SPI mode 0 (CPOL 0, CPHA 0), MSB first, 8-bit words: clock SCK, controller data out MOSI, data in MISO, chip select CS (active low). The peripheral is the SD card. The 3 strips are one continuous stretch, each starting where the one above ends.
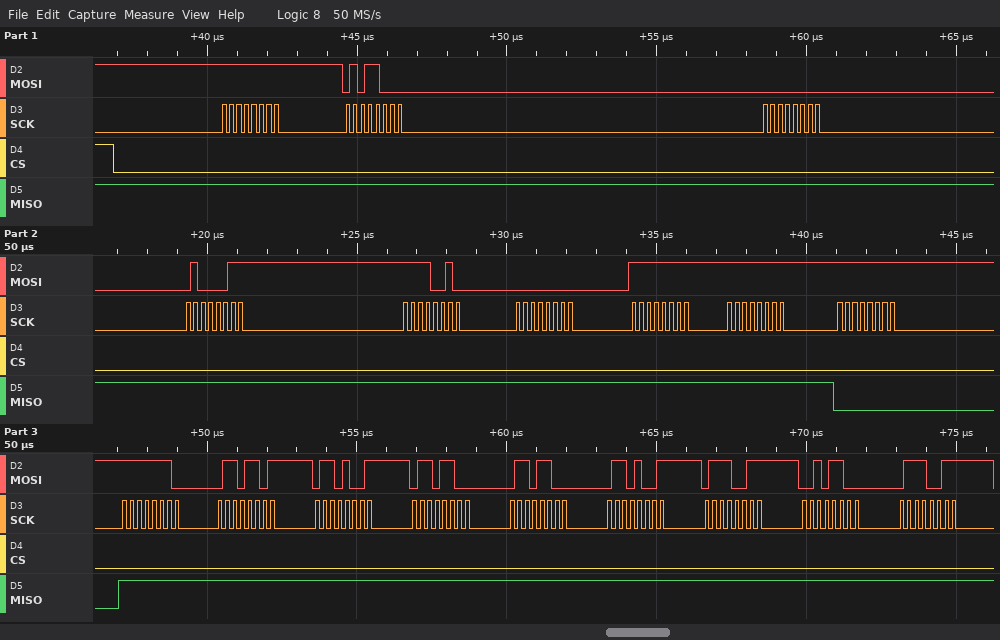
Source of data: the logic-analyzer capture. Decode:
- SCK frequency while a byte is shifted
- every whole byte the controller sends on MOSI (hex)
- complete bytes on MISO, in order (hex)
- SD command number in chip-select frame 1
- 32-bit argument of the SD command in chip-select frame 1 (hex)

4 MHz
FF 58 00 43 F2 00 FF FF FF FE 6D 69 6C 6C 69 73 2C 73
FF FF FF FF FF FF FF FF 00 FF FF FF FF FF FF FF FF FF
CMD24
0x0043F200
